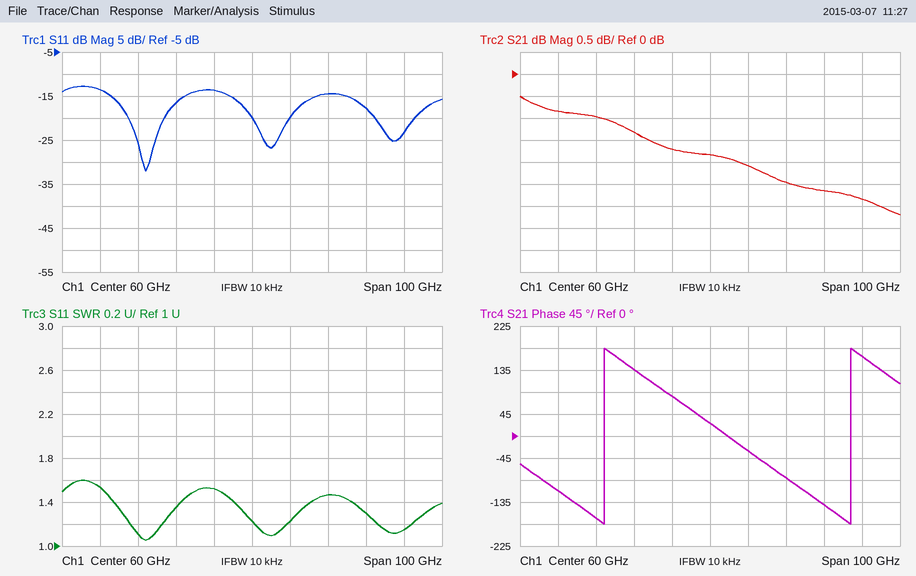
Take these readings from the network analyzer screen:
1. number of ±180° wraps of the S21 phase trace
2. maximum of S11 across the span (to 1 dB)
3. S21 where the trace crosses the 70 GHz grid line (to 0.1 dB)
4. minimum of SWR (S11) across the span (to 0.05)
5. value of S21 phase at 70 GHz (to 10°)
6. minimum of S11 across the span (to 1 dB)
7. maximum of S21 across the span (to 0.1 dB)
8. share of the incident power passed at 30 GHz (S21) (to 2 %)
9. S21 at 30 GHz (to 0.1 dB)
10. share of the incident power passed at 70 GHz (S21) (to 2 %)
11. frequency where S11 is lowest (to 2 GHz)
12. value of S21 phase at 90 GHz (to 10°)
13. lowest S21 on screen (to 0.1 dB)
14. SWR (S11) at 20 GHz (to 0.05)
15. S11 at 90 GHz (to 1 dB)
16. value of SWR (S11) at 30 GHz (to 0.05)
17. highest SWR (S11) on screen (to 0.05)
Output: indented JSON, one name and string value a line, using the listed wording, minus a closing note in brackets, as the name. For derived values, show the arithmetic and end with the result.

{
  "number of ±180° wraps of the S21 phase trace": "2",
  "maximum of S11 across the span": "-13 dB",
  "S21 where the trace crosses the 70 GHz grid line": "-2.1 dB",
  "minimum of SWR (S11) across the span": "1.05",
  "value of S21 phase at 70 GHz": "-30°",
  "minimum of S11 across the span": "-32 dB",
  "maximum of S21 across the span": "-0.5 dB",
  "share of the incident power passed at 30 GHz (S21)": "10^(-1/10) ≈ 79.4 %, so 80 % to the nearest 2 %",
  "S21 at 30 GHz": "-1.0 dB",
  "share of the incident power passed at 70 GHz (S21)": "10^(-2.1/10) ≈ 62 %",
  "frequency where S11 is lowest": "32 GHz",
  "value of S21 phase at 90 GHz": "-140°",
  "lowest S21 on screen": "-3.2 dB",
  "SWR (S11) at 20 GHz": "1.55",
  "S11 at 90 GHz": "-18 dB",
  "value of SWR (S11) at 30 GHz": "1.10",
  "highest SWR (S11) on screen": "1.60"
}
